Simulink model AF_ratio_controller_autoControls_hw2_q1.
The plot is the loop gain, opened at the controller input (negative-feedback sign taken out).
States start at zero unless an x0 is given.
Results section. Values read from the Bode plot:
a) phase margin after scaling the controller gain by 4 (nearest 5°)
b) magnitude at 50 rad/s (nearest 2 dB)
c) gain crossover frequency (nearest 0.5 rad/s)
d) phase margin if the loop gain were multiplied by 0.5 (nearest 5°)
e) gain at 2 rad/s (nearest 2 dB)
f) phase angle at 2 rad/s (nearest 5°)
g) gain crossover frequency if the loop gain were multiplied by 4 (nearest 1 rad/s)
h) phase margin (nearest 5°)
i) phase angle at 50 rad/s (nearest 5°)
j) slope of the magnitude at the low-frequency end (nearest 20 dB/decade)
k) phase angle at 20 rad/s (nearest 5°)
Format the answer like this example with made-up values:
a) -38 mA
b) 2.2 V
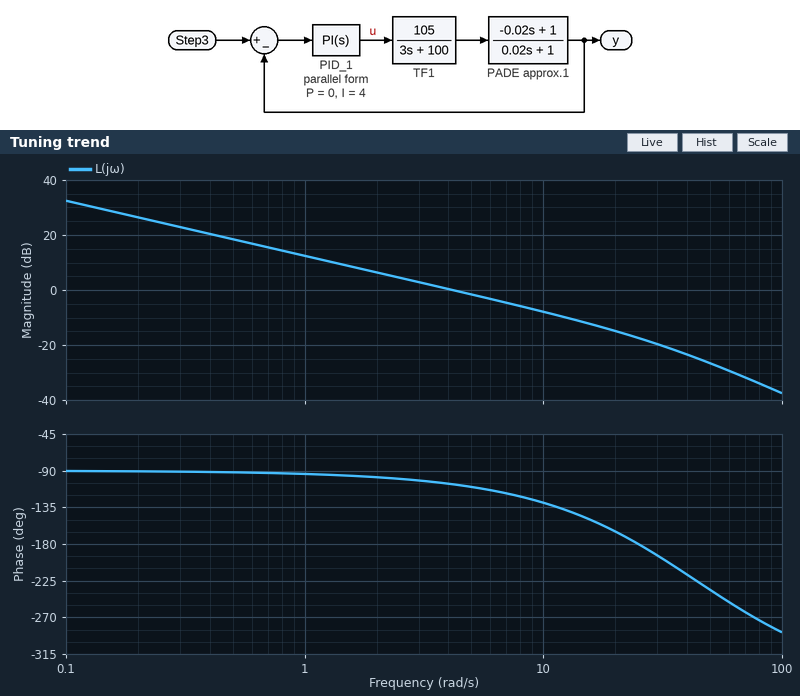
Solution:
a) 30°
b) -26 dB
c) 4.0 rad/s
d) 80°
e) 6 dB
f) -100°
g) 15 rad/s
h) 75°
i) -235°
j) -20 dB/decade
k) -165°
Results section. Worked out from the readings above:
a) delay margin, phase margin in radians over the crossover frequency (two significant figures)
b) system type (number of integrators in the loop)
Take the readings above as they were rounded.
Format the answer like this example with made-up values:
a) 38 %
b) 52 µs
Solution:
a) 0.33 s
b) 1
